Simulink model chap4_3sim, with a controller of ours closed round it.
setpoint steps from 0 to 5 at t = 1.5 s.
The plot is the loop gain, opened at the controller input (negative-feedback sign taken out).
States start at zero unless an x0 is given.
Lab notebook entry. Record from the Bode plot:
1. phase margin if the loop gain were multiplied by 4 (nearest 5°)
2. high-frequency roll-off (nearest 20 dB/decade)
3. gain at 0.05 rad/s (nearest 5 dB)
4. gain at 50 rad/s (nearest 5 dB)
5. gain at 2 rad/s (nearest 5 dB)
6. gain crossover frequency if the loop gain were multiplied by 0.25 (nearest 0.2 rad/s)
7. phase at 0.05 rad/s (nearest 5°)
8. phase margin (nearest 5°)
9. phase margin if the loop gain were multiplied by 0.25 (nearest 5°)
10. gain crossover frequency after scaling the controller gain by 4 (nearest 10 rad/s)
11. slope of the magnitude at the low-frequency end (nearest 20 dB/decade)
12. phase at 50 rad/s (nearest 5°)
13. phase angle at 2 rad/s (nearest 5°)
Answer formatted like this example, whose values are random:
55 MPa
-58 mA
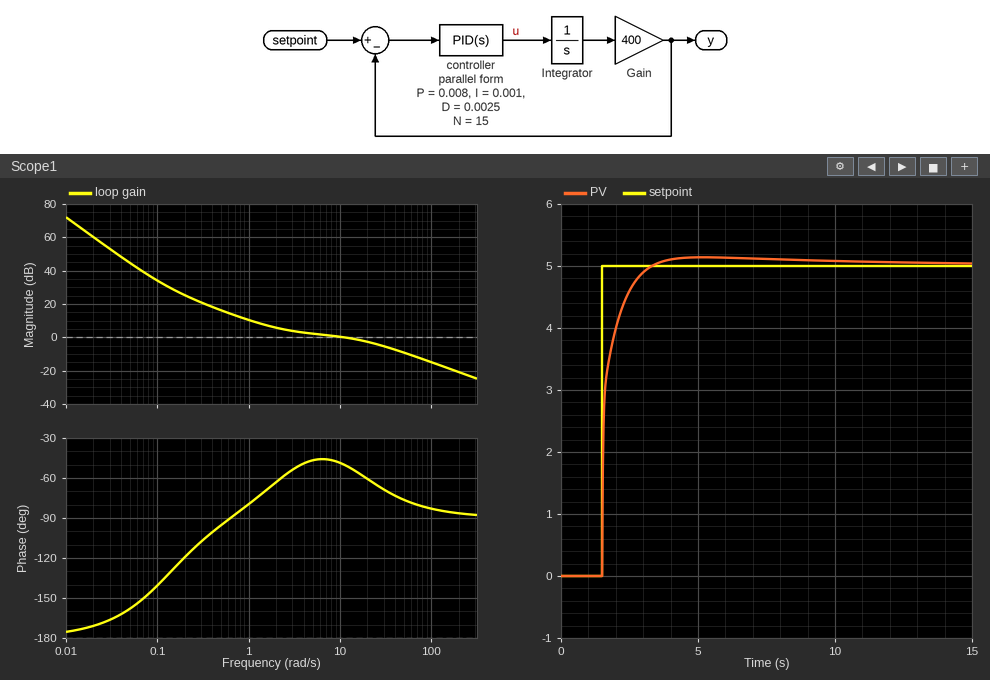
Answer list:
100°
-20 dB/decade
45 dB
-10 dB
5 dB
0.8 rad/s
-160°
130°
95°
70 rad/s
-40 dB/decade
-75°
-65°
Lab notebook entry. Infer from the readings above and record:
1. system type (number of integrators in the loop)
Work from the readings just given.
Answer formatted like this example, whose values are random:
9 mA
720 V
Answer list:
2
